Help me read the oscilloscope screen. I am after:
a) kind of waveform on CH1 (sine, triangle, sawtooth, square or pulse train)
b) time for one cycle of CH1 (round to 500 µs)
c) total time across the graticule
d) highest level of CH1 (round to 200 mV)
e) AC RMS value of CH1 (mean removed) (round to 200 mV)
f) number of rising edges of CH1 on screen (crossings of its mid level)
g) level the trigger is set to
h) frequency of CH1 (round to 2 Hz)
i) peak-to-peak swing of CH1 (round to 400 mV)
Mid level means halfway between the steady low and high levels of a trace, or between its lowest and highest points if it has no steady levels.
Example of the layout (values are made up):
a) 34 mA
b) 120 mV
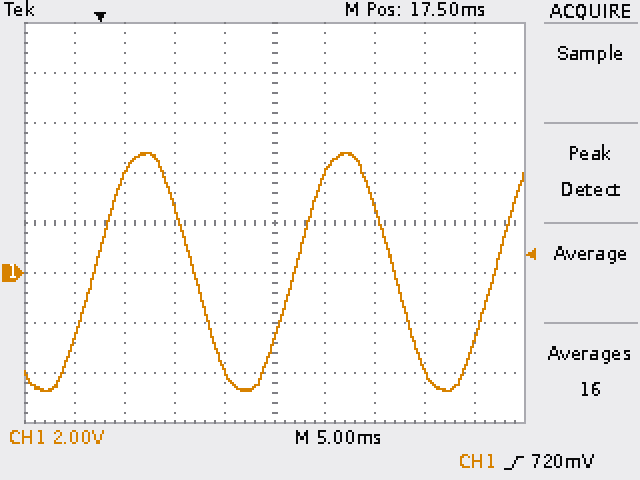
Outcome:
a) sine
b) 20.0 ms
c) 50 ms
d) 4.8 V
e) 3.4 V
f) 3
g) 720 mV
h) 50 Hz
i) 9.6 V
